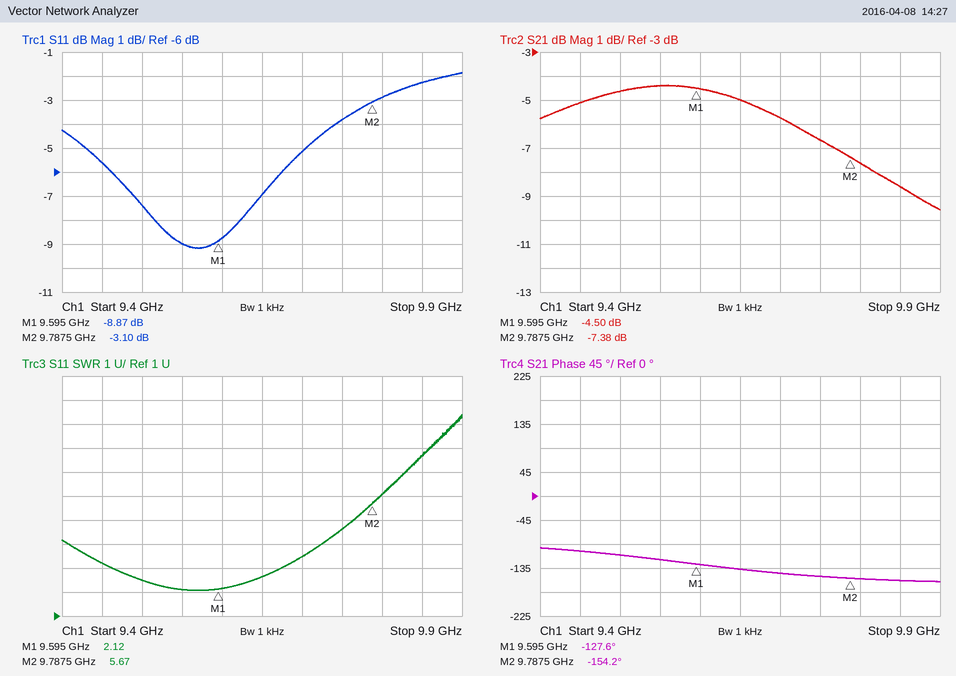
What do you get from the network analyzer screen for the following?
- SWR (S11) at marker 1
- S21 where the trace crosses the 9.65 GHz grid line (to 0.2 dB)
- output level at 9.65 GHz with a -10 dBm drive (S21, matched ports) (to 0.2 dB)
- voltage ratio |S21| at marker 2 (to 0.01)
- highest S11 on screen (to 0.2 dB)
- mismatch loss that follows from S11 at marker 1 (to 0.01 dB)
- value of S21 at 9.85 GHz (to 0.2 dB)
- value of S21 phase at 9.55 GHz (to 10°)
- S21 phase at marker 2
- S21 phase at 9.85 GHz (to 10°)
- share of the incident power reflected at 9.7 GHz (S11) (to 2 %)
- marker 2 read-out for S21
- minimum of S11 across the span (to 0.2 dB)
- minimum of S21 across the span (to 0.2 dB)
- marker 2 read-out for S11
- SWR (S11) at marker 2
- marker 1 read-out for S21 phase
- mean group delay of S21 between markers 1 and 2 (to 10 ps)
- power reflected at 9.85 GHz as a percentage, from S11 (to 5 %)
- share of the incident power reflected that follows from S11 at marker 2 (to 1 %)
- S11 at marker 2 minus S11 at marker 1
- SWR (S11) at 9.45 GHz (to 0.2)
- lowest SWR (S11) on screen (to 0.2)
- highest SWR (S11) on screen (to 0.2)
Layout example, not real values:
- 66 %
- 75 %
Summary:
- 2.12
- -5.0 dB
- -15.0 dBm
- 0.43
- -1.8 dB
- 0.60 dB
- -8.6 dB
- -120°
- -154.2°
- -160°
- 30 %
- -7.38 dB
- -9.2 dB
- -9.6 dB
- -3.10 dB
- 5.67
- -127.6°
- 380 ps
- 60 %
- 49 %
- 5.77 dB
- 3.2
- 2.0
- 9.4
